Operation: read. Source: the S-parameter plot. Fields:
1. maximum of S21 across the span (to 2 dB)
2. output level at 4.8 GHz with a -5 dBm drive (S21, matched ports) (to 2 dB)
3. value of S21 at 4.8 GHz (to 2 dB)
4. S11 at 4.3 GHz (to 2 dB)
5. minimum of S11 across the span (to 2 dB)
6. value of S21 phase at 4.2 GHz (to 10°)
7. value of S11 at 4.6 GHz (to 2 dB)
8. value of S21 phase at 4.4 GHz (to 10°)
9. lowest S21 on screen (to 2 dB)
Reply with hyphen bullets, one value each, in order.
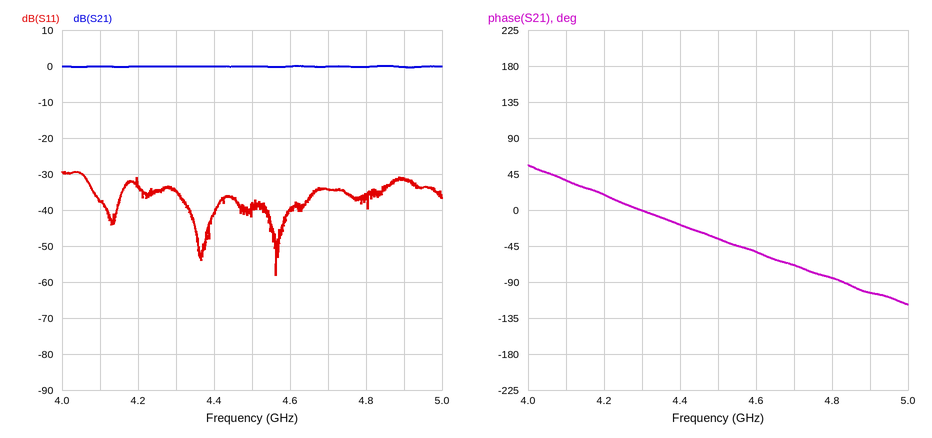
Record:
- 0 dB
- -6 dBm
- 0 dB
- -34 dB
- -58 dB
- 20°
- -40 dB
- -20°
- 0 dB
